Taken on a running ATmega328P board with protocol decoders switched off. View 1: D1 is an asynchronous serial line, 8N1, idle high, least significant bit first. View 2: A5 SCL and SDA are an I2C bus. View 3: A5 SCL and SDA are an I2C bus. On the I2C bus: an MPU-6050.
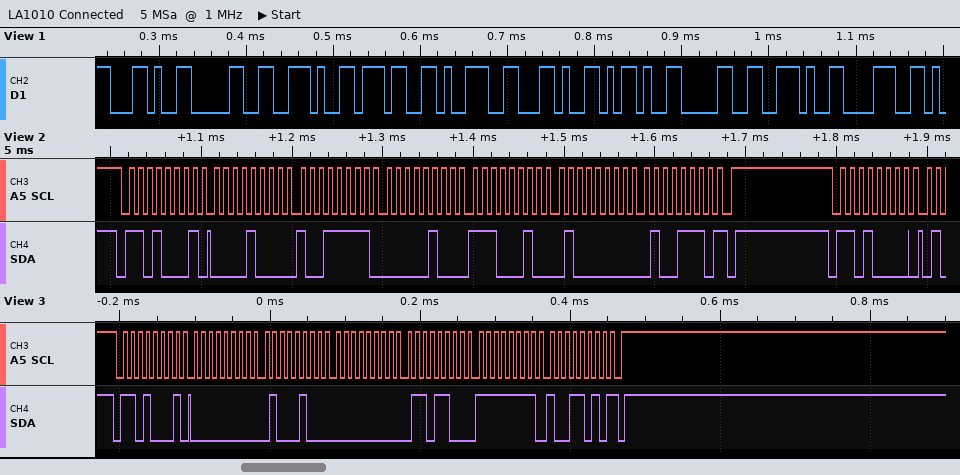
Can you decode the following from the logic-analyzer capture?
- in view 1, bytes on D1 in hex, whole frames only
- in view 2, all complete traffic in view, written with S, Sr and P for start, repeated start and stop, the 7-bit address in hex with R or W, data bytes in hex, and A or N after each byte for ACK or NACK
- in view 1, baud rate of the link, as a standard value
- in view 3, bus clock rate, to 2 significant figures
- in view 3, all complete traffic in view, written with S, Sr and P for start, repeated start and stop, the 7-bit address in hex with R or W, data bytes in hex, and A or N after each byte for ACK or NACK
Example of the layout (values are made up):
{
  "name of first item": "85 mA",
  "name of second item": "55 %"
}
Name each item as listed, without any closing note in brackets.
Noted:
{
  "in view 1, bytes on D1 in hex, whole frames only": "0x2C 0x30 0x2E 0x37 0x39 0x2C 0x2D 0x30 0x2E 0x38",
  "in view 2, all complete traffic in view, written with S, Sr and P for start, repeated start and stop, the 7-bit address in hex with R or W, data bytes in hex, and A or N after each byte for ACK or NACK": "S 68R A 08 A 9F A 04 A E2 A 40 A 4E N P S 68W A",
  "in view 1, baud rate of the link, as a standard value": "115200 baud",
  "in view 3, bus clock rate, to 2 significant figures": "100 kHz",
  "in view 3, all complete traffic in view, written with S, Sr and P for start, repeated start and stop, the 7-bit address in hex with R or W, data bytes in hex, and A or N after each byte for ACK or NACK": "S 68R A 00 A 44 A 00 A 6C A FF A 9A N P"
}
